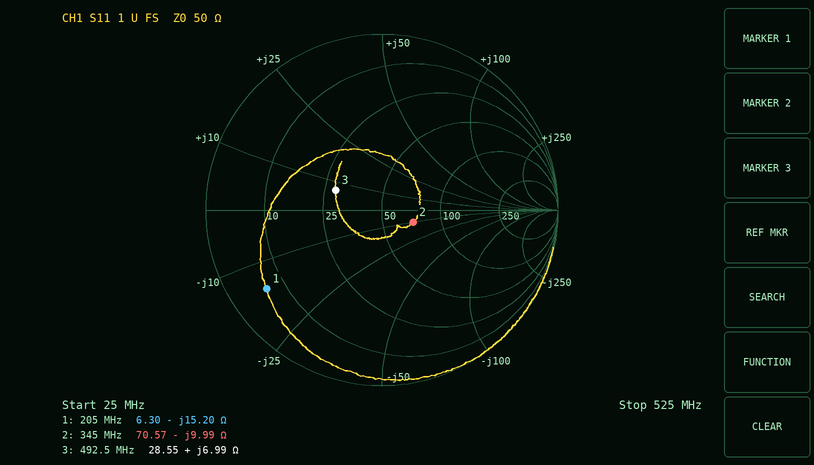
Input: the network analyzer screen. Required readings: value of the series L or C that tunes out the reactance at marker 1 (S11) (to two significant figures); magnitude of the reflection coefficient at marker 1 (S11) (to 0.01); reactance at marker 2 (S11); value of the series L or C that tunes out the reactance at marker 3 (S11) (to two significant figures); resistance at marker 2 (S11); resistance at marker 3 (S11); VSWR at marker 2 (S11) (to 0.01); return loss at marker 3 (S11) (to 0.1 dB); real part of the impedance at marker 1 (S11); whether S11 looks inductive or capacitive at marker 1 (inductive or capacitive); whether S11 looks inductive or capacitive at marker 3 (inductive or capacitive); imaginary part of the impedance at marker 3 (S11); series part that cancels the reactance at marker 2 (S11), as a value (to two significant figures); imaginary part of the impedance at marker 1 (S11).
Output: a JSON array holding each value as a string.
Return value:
["12 nH", "0.79", "-9.99 Ω", "46 pF", "70.57 Ω", "28.55 Ω", "1.47", "10.9 dB", "6.30 Ω", "capacitive", "inductive", "+6.99 Ω", "4.6 nH", "-15.20 Ω"]
